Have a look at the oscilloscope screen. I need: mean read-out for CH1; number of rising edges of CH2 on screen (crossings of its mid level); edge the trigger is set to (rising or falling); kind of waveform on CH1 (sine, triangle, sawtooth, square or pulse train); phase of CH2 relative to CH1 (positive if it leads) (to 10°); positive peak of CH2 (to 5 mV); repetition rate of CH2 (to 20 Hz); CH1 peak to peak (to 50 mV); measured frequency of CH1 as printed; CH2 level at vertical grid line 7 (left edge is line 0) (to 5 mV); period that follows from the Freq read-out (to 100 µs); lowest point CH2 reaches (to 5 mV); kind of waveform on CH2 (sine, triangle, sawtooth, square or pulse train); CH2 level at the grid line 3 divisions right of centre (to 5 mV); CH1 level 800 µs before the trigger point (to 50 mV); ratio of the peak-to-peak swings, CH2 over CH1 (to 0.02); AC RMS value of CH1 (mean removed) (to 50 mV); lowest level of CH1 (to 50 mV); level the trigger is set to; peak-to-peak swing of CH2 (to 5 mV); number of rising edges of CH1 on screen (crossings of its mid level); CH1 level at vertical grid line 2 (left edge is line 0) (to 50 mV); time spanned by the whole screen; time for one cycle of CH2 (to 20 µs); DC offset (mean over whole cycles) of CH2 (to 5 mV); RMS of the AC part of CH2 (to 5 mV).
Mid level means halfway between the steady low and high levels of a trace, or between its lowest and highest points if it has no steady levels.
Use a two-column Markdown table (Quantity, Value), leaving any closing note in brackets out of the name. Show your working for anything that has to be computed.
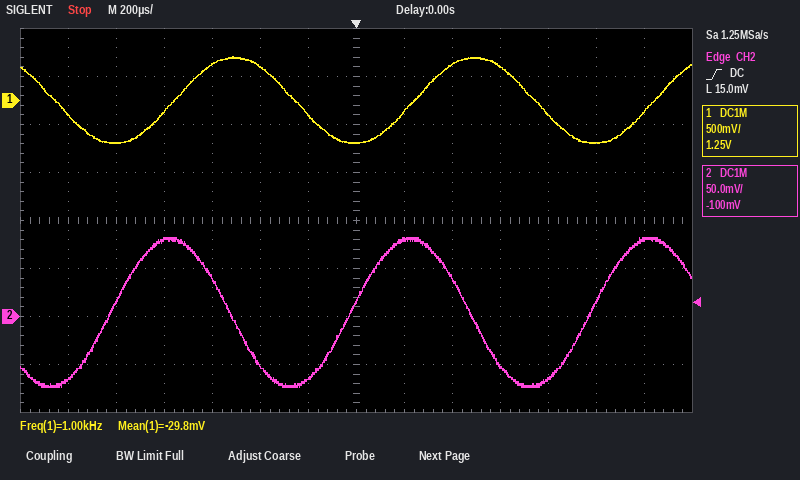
| Quantity | Value |
|---|---|
| mean read-out for CH1 | -29.8 mV |
| number of rising edges of CH2 on screen | 3 |
| edge the trigger is set to | rising |
| kind of waveform on CH1 | sine |
| phase of CH2 relative to CH1 (positive if it leads) | +100° |
| positive peak of CH2 | 80 mV |
| repetition rate of CH2 | 1 / 1.00 ms ≈ 1.00 kHz |
| CH1 peak to peak | 450 mV − (-450 mV) = 900 mV |
| measured frequency of CH1 as printed | 1.00 kHz |
| CH2 level at vertical grid line 7 (left edge is line 0) | 15 mV |
| period that follows from the Freq read-out | 1 / 1.00 kHz ≈ 1.0 ms |
| lowest point CH2 reaches | -75 mV |
| kind of waveform on CH2 | sine |
| CH2 level at the grid line 3 divisions right of centre | -50 mV |
| CH1 level 800 µs before the trigger point | -100 mV |
| ratio of the peak-to-peak swings, CH2 over CH1 | 155 mV / 900 mV ≈ 0.172, so 0.18 to the nearest 0.02 |
| AC RMS value of CH1 (mean removed) | 900 mV / (2√2) ≈ 318 mV, so 300 mV to the nearest 50 mV |
| lowest level of CH1 | -450 mV |
| level the trigger is set to | 15.0 mV |
| peak-to-peak swing of CH2 | 80 mV − (-75 mV) = 155 mV |
| number of rising edges of CH1 on screen | 3 |
| CH1 level at vertical grid line 2 (left edge is line 0) | -450 mV |
| time spanned by the whole screen | 2.8 ms |
| time for one cycle of CH2 | 1.00 ms |
| DC offset (mean over whole cycles) of CH2 | (80 mV + (-75 mV)) / 2 ≈ 2.50 mV, so 5 mV to the nearest 5 mV |
| RMS of the AC part of CH2 | 155 mV / (2√2) ≈ 55 mV |
